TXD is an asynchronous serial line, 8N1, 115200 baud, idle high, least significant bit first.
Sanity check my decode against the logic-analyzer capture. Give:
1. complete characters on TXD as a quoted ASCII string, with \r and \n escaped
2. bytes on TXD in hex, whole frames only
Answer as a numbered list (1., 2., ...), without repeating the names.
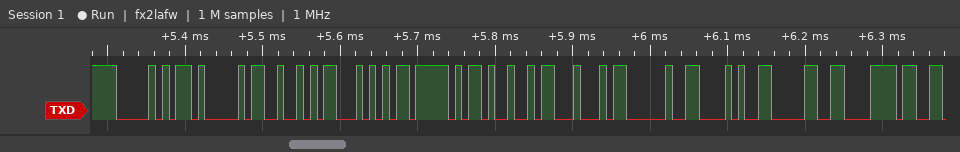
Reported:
1. "PART_ID (0x"
2. 0x50 0x41 0x52 0x54 0x5F 0x49 0x44 0x20 0x28 0x30 0x78
